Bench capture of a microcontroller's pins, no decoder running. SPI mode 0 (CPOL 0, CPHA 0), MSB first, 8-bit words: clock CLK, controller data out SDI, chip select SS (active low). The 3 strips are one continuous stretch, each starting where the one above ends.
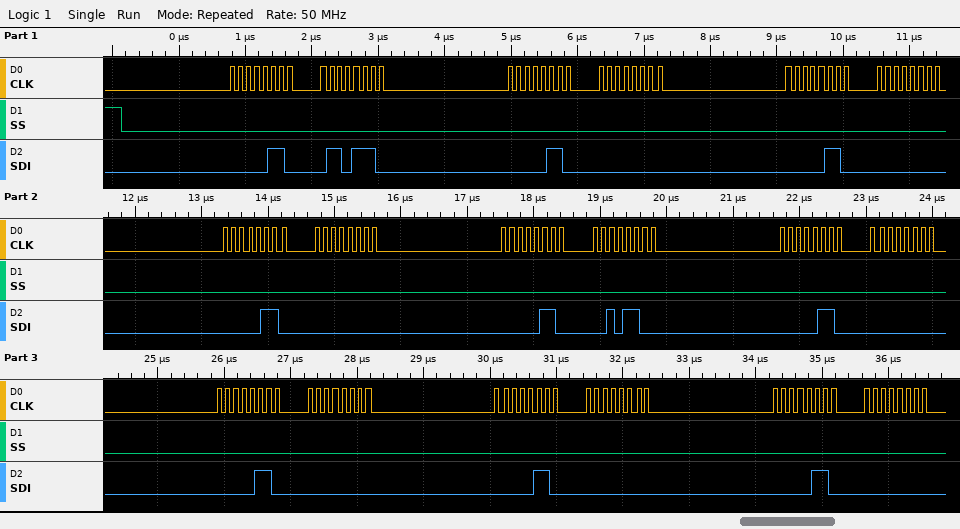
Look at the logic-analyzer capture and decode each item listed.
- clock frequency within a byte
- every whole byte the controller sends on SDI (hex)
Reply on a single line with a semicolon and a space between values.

8 MHz; 0x06 0x6E 0x06 0x00 0x06 0x00 0x06 0x00 0x06 0x2C 0x06 0x00 0x06 0x00 0x06 0x00 0x06 0x00
